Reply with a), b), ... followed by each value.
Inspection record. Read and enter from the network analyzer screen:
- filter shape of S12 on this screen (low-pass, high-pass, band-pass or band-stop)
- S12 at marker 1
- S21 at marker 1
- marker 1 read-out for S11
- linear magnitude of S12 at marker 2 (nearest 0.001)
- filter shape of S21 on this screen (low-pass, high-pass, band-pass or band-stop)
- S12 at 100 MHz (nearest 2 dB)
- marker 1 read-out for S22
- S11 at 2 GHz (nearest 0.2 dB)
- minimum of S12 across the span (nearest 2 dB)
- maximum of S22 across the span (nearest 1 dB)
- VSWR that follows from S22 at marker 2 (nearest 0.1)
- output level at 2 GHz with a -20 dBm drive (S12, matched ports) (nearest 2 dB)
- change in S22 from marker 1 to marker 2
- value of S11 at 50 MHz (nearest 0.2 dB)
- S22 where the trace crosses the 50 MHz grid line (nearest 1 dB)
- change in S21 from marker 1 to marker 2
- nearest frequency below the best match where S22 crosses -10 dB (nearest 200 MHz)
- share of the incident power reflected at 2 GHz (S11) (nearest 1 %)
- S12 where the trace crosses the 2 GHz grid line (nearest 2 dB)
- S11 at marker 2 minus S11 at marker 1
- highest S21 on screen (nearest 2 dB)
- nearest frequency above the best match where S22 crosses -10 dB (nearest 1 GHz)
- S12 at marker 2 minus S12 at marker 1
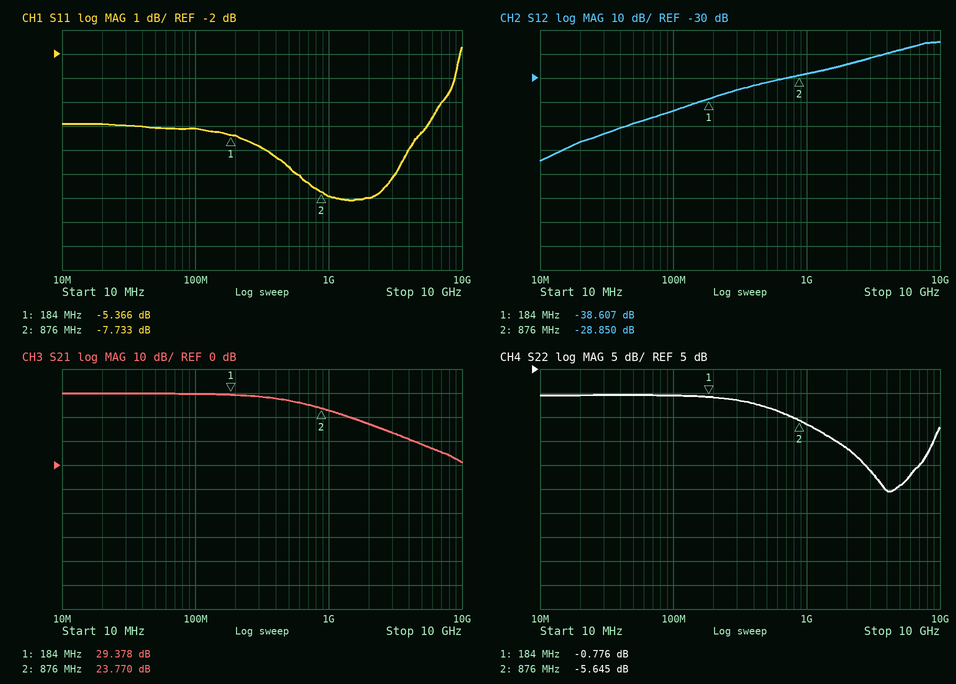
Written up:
a) high-pass
b) -38.607 dB
c) 29.378 dB
d) -5.366 dB
e) 0.036
f) low-pass
g) -44 dB
h) -0.776 dB
i) -8.0 dB
j) -64 dB
k) 0 dB
l) 3.2
m) -44 dBm
n) -4.869 dB
o) -5.0 dB
p) 0 dB
q) -5.608 dB
r) 1.6 GHz
s) 16 %
t) -24 dB
u) -2.367 dB
v) 30 dB
w) 9 GHz
x) 9.757 dB
